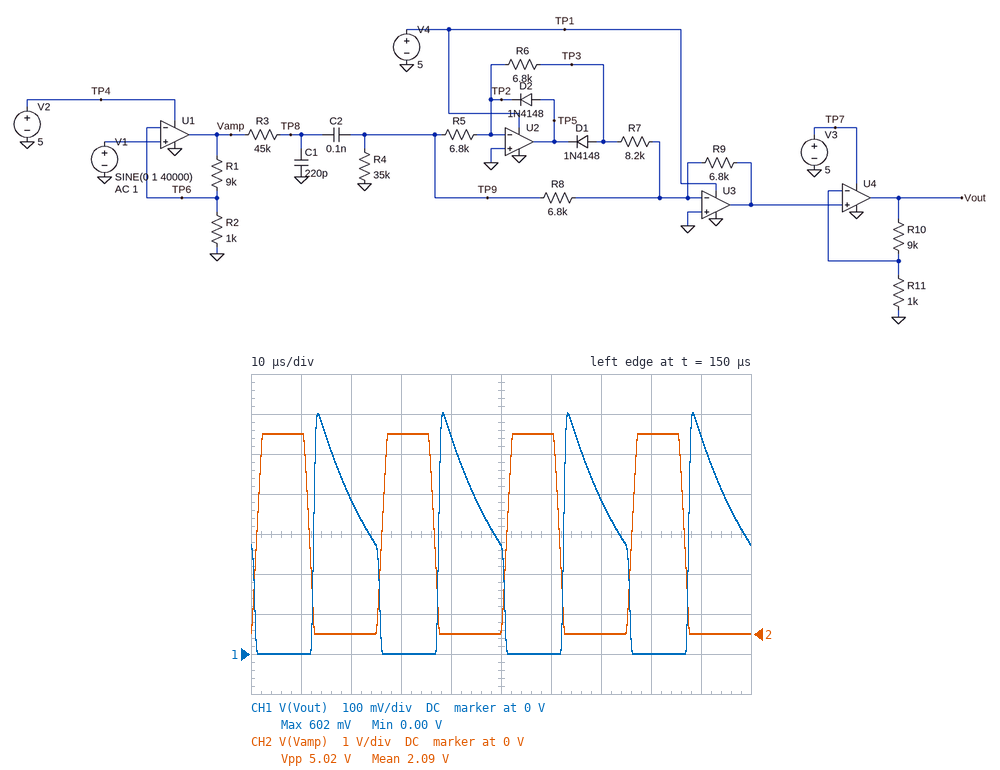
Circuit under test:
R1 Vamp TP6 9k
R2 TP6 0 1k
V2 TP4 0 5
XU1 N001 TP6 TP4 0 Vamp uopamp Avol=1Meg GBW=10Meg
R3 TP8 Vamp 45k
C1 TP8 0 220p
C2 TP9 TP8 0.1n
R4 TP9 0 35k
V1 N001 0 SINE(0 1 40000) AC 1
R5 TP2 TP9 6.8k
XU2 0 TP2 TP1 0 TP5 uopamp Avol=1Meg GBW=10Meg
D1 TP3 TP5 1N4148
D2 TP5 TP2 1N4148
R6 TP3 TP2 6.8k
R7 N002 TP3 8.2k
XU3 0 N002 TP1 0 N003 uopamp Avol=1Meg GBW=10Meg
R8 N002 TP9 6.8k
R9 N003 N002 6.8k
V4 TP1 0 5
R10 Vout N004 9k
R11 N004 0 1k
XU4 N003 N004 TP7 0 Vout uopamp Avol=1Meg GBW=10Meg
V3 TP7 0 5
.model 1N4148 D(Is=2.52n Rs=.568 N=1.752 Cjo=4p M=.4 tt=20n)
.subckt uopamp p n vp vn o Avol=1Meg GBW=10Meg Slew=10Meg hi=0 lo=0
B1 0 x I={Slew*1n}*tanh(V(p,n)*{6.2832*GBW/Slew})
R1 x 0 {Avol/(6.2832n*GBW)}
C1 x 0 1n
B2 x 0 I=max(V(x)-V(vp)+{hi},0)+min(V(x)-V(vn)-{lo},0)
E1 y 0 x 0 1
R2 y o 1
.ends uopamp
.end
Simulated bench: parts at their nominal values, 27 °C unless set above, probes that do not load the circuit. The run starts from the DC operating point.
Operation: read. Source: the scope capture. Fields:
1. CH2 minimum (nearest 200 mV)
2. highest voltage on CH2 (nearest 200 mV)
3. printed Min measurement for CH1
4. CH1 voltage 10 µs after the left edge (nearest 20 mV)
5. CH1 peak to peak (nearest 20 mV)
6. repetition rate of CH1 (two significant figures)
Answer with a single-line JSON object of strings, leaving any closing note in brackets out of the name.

{"CH2 minimum": "0 V", "highest voltage on CH2": "5.0 V", "printed Min measurement for CH1": "0.00 V", "CH1 voltage 10 µs after the left edge": "0 V", "CH1 peak to peak": "600 mV", "repetition rate of CH1": "40 kHz"}
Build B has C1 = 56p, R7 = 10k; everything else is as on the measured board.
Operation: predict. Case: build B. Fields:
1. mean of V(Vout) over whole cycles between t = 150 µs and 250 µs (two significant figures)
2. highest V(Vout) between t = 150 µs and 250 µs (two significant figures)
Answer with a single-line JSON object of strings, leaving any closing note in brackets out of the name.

{"mean of V(Vout) over whole cycles between t = 150 µs and 250 µs": "390 mV", "highest V(Vout) between t = 150 µs and 250 µs": "1.4 V"}
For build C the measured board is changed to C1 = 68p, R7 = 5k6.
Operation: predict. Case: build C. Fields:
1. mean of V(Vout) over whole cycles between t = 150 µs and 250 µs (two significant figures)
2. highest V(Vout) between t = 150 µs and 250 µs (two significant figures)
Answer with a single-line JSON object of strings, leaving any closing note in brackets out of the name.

{"mean of V(Vout) over whole cycles between t = 150 µs and 250 µs": "370 mV", "highest V(Vout) between t = 150 µs and 250 µs": "1.3 V"}
